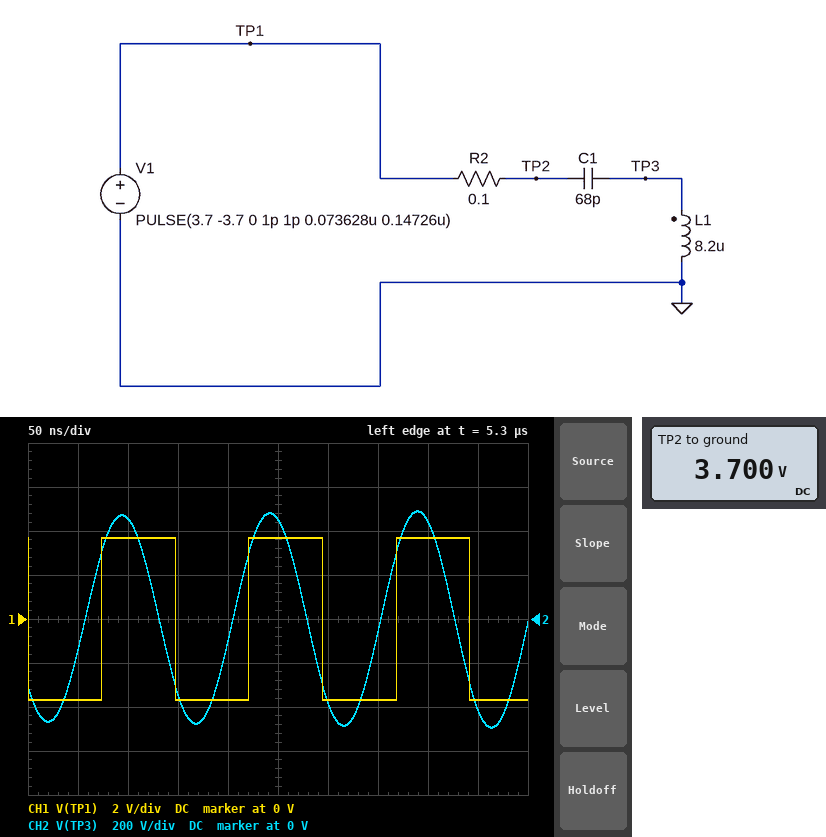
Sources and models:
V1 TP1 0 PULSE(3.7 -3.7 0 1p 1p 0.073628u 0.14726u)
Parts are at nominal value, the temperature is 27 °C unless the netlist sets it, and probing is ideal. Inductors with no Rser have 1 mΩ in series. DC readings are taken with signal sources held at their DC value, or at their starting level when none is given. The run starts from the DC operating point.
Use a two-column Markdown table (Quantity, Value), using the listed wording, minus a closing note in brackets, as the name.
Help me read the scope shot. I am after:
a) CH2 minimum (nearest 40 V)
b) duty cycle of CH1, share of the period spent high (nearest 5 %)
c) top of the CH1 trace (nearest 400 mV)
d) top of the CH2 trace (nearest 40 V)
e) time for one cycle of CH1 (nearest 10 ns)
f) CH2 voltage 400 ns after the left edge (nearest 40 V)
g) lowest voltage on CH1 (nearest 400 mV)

| Quantity | Value |
|---|---|
| CH2 minimum | -480 V |
| duty cycle of CH1, share of the period spent high | 50 % |
| top of the CH1 trace | 3.6 V |
| top of the CH2 trace | 480 V |
| time for one cycle of CH1 | 150 ns |
| CH2 voltage 400 ns after the left edge | 440 V |
| lowest voltage on CH1 | -3.6 V |
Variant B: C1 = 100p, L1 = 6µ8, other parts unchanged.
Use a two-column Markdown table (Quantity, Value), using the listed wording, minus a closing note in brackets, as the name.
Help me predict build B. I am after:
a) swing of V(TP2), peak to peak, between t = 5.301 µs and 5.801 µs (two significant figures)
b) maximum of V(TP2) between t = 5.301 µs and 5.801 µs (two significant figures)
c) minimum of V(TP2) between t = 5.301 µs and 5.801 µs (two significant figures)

| Quantity | Value |
|---|---|
| swing of V(TP2), peak to peak, between t = 5.301 µs and 5.801 µs | 7.4 V |
| maximum of V(TP2) between t = 5.301 µs and 5.801 µs | 3.7 V |
| minimum of V(TP2) between t = 5.301 µs and 5.801 µs | -3.7 V |
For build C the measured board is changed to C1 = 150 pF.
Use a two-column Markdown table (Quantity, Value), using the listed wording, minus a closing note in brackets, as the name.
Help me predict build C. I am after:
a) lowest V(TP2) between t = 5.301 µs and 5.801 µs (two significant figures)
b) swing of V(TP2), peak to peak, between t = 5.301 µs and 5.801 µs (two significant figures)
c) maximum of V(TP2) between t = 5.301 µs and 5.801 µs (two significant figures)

| Quantity | Value |
|---|---|
| lowest V(TP2) between t = 5.301 µs and 5.801 µs | -3.7 V |
| swing of V(TP2), peak to peak, between t = 5.301 µs and 5.801 µs | 7.4 V |
| maximum of V(TP2) between t = 5.301 µs and 5.801 µs | 3.7 V |
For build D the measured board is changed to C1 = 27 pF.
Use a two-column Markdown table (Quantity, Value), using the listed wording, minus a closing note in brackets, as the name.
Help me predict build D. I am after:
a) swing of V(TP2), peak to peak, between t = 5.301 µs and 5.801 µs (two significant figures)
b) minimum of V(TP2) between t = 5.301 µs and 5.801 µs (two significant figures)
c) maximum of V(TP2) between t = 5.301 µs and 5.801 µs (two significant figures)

| Quantity | Value |
|---|---|
| swing of V(TP2), peak to peak, between t = 5.301 µs and 5.801 µs | 7.4 V |
| minimum of V(TP2) between t = 5.301 µs and 5.801 µs | -3.7 V |
| maximum of V(TP2) between t = 5.301 µs and 5.801 µs | 3.7 V |
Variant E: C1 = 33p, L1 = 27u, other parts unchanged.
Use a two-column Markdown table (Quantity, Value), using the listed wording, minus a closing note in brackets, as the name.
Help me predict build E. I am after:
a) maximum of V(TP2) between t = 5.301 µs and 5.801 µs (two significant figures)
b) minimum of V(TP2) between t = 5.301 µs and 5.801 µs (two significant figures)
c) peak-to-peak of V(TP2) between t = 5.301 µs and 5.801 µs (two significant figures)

| Quantity | Value |
|---|---|
| maximum of V(TP2) between t = 5.301 µs and 5.801 µs | 3.7 V |
| minimum of V(TP2) between t = 5.301 µs and 5.801 µs | -3.7 V |
| peak-to-peak of V(TP2) between t = 5.301 µs and 5.801 µs | 7.4 V |
